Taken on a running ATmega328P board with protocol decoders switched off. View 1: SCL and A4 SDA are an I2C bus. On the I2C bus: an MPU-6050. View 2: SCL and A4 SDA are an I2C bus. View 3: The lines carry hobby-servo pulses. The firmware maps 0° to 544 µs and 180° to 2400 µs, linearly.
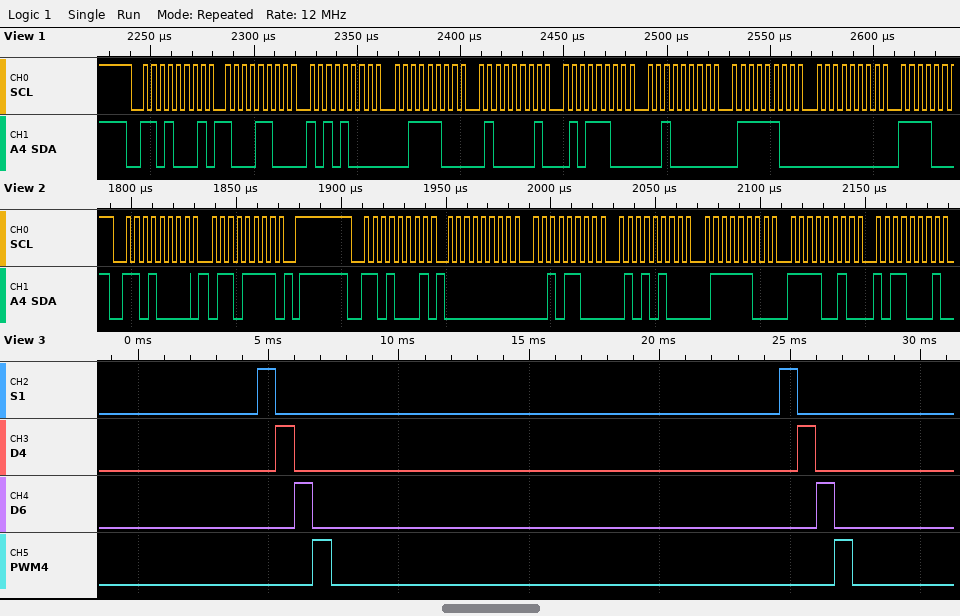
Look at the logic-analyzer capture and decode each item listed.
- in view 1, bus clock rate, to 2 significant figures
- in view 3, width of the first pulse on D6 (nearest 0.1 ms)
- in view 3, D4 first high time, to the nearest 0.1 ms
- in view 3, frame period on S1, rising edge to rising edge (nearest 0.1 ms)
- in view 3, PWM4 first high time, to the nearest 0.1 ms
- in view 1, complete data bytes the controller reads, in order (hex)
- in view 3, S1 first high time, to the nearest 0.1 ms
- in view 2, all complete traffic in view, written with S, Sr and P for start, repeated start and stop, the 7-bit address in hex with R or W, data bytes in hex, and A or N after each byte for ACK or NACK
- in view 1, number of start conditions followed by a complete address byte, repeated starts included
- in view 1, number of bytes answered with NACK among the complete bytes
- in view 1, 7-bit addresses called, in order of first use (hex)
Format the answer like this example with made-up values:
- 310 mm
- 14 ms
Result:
- 250 kHz
- 0.7 ms
- 0.7 ms
- 20.0 ms
- 0.7 ms
- 8C A8 3C 41 5C 20 7C 00
- 0.7 ms
- S 68W A 6F A P S 68R A 00 A 2C A 54 A 7C A F2 A B1 A
- 1
- 0
- 0x68
